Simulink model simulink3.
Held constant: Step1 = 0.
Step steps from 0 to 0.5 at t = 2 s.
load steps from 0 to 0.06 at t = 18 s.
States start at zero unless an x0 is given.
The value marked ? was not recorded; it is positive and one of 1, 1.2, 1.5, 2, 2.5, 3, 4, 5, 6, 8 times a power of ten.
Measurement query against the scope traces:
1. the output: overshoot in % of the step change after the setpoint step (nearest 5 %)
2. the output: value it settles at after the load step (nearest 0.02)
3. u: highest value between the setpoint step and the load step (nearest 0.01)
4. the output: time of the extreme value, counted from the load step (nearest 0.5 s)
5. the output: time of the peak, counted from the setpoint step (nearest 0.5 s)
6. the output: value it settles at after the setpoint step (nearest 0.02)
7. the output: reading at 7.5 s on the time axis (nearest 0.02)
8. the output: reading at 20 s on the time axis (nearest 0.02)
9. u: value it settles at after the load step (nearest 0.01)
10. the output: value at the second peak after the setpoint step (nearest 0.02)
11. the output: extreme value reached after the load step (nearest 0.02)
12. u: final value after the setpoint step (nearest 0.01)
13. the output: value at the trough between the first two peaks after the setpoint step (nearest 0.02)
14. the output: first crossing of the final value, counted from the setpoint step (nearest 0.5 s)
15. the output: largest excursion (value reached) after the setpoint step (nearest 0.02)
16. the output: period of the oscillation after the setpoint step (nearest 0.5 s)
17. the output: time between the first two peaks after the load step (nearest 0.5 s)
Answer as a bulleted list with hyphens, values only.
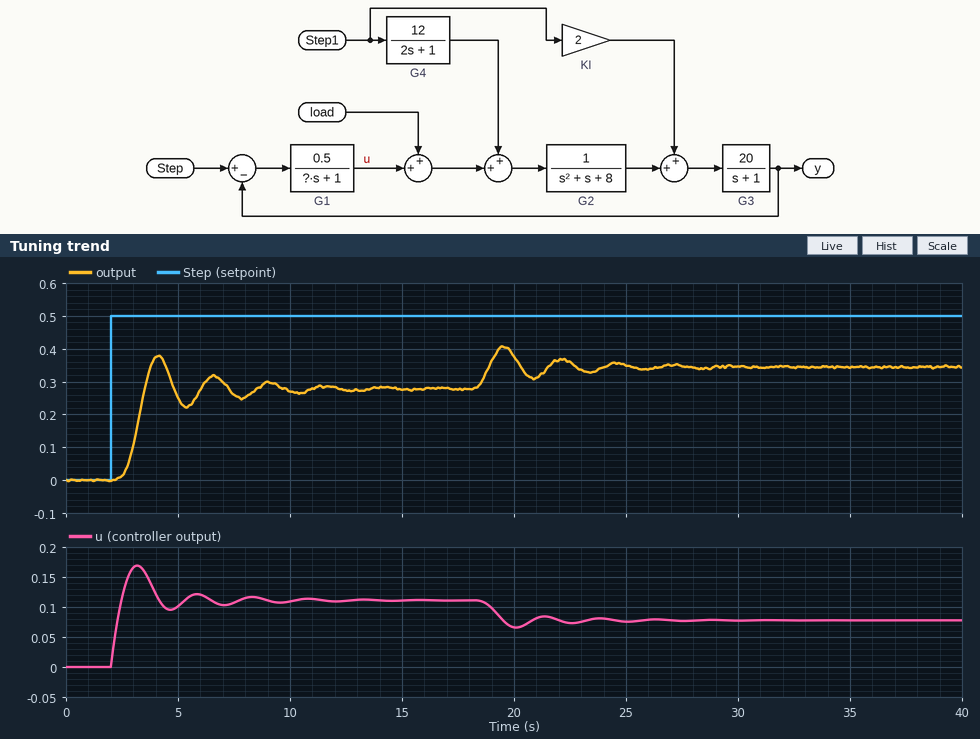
- 35 %
- 0.34
- 0.17
- 1.5 s
- 2.0 s
- 0.28
- 0.26
- 0.38
- 0.08
- 0.32
- 0.40
- 0.11
- 0.22
- 1.5 s
- 0.38
- 2.5 s
- 2.5 s
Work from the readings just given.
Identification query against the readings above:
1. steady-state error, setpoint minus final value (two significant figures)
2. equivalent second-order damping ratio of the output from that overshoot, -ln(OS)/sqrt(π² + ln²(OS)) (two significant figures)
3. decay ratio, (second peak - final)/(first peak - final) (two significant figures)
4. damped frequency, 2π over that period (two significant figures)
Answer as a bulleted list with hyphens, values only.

- 0.22
- 0.32
- 0.40
- 2.5 rad/s
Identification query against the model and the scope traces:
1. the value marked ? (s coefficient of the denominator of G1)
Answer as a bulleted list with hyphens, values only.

- 0.8
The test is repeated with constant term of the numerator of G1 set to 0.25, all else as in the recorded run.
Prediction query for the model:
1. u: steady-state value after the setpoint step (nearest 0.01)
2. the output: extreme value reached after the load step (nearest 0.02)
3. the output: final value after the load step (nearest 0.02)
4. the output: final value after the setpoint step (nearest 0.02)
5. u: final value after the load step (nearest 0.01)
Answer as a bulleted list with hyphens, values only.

- 0.08
- 0.32
- 0.28
- 0.20
- 0.05
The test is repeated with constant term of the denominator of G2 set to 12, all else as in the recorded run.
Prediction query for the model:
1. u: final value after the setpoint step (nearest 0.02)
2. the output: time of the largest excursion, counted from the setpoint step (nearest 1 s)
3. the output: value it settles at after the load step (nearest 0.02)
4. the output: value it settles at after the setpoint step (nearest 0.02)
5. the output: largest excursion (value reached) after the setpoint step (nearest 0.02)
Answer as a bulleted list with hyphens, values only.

- 0.14
- 4 s
- 0.28
- 0.22
- 0.24
